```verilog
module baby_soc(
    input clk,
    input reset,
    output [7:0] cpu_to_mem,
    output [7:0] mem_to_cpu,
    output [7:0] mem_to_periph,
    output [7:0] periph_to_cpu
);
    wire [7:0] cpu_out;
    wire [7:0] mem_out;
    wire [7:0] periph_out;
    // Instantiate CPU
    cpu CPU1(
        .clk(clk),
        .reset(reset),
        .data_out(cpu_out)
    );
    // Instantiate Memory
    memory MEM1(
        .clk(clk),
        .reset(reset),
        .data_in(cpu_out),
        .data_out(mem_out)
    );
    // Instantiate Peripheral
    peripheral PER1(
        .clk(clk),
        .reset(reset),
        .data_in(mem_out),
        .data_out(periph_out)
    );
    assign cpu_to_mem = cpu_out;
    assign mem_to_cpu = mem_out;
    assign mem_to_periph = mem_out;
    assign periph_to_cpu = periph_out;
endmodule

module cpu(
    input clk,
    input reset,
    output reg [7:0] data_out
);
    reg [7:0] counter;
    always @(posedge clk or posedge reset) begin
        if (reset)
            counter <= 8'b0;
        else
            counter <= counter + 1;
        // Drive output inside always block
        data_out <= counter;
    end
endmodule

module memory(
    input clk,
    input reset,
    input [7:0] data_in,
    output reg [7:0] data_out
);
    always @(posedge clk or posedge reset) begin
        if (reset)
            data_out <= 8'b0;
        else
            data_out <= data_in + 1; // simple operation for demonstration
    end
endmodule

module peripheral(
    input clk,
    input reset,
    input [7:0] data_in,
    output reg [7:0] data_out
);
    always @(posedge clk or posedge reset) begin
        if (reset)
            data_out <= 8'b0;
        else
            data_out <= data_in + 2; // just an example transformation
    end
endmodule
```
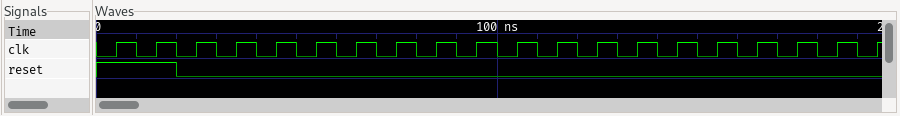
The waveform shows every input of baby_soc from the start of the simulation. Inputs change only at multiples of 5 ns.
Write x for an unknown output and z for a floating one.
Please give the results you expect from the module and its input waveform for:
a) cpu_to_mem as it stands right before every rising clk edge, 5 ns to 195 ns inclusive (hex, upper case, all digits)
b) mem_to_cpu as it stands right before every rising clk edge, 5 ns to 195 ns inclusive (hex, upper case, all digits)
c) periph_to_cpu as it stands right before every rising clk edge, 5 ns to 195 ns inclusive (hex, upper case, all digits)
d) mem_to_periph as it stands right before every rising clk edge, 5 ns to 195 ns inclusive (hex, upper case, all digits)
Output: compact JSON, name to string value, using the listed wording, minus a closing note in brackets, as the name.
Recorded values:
{"cpu_to_mem as it stands right before every rising clk edge, 5 ns to 195 ns inclusive": "x, 00, 00, 00, 01, 02, 03, 04, 05, 06, 07, 08, 09, 0A, 0B, 0C, 0D, 0E, 0F, 10", "mem_to_cpu as it stands right before every rising clk edge, 5 ns to 195 ns inclusive": "00, 00, 00, 01, 01, 02, 03, 04, 05, 06, 07, 08, 09, 0A, 0B, 0C, 0D, 0E, 0F, 10", "periph_to_cpu as it stands right before every rising clk edge, 5 ns to 195 ns inclusive": "00, 00, 00, 02, 03, 03, 04, 05, 06, 07, 08, 09, 0A, 0B, 0C, 0D, 0E, 0F, 10, 11", "mem_to_periph as it stands right before every rising clk edge, 5 ns to 195 ns inclusive": "00, 00, 00, 01, 01, 02, 03, 04, 05, 06, 07, 08, 09, 0A, 0B, 0C, 0D, 0E, 0F, 10"}
